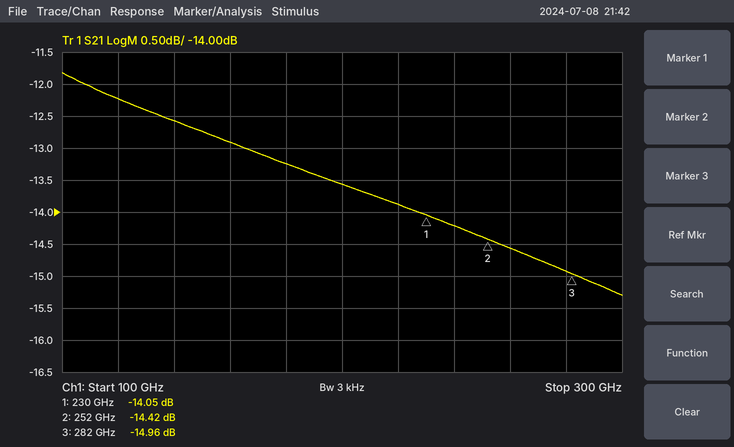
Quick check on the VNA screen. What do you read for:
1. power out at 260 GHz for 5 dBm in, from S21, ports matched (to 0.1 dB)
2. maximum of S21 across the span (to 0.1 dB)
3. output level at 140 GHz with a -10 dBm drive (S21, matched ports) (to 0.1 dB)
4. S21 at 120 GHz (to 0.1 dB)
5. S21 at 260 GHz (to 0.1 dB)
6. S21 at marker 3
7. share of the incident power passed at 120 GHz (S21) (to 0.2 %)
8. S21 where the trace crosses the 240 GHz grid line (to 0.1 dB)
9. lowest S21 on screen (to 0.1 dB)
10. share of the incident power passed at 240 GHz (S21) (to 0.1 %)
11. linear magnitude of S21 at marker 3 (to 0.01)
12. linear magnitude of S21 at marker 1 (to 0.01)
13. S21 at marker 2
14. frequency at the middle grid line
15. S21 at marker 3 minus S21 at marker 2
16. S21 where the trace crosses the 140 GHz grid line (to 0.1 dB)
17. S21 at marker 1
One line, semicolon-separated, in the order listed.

-9.6 dBm; -11.8 dB; -22.6 dBm; -12.2 dB; -14.6 dB; -14.96 dB; 6.0 %; -14.2 dB; -15.3 dB; 3.8 %; 0.18; 0.20; -14.42 dB; 200 GHz; -0.54 dB; -12.6 dB; -14.05 dB
